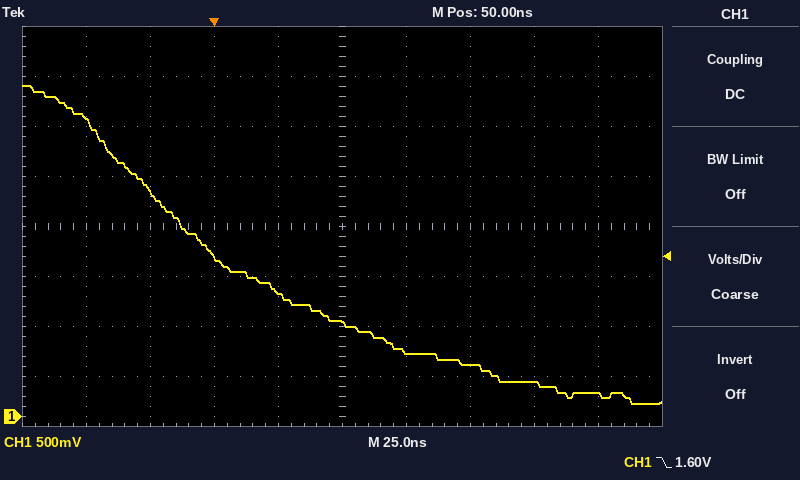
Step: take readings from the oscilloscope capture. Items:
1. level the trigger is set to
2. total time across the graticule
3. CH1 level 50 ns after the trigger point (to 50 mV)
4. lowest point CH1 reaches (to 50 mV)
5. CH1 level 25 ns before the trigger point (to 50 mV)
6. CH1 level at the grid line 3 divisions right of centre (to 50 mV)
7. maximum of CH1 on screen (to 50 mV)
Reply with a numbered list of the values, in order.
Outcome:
1. 1.60 V
2. 250 ns
3. 950 mV
4. 150 mV
5. 2.25 V
6. 350 mV
7. 3.30 V
